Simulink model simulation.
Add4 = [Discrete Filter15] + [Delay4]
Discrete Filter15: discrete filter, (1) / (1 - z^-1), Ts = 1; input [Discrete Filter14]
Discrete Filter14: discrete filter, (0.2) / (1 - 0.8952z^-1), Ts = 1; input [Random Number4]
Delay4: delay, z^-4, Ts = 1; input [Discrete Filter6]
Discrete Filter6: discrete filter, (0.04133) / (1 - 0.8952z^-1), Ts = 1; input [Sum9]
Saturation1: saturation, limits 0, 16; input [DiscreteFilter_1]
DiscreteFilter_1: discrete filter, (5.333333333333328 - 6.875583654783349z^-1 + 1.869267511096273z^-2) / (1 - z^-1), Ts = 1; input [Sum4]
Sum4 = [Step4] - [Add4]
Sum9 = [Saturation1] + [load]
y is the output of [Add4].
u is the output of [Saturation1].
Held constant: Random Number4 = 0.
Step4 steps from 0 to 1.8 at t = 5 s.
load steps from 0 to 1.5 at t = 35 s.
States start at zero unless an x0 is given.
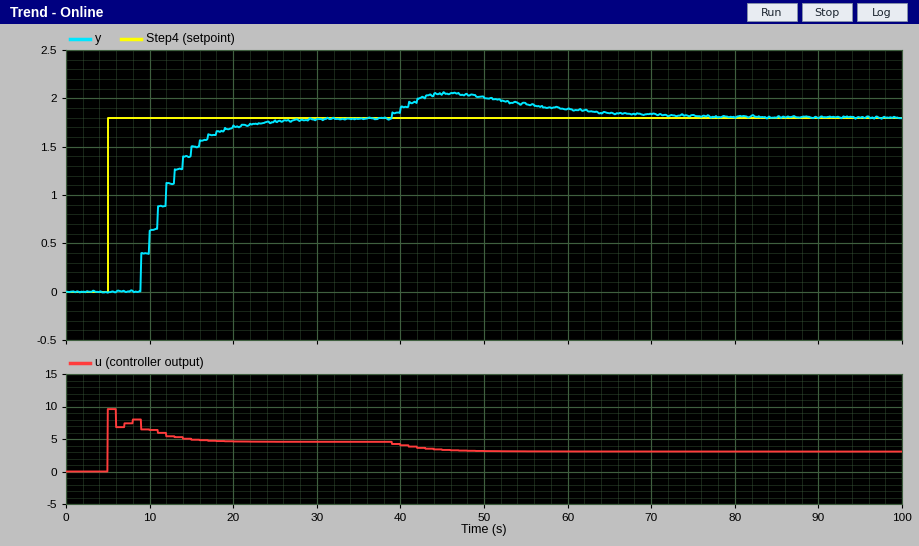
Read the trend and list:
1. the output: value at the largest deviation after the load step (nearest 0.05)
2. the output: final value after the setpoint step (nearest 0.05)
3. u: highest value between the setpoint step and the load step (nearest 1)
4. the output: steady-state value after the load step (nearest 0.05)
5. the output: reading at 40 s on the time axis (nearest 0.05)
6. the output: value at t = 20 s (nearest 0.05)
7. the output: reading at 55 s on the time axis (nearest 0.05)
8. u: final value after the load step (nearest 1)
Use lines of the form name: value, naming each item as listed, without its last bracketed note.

the output: value at the largest deviation after the load step: 2.05
the output: final value after the setpoint step: 1.80
u: highest value between the setpoint step and the load step: 10
the output: steady-state value after the load step: 1.80
the output: reading at 40 s on the time axis: 1.90
the output: value at t = 20 s: 1.70
the output: reading at 55 s on the time axis: 1.95
u: final value after the load step: 3
